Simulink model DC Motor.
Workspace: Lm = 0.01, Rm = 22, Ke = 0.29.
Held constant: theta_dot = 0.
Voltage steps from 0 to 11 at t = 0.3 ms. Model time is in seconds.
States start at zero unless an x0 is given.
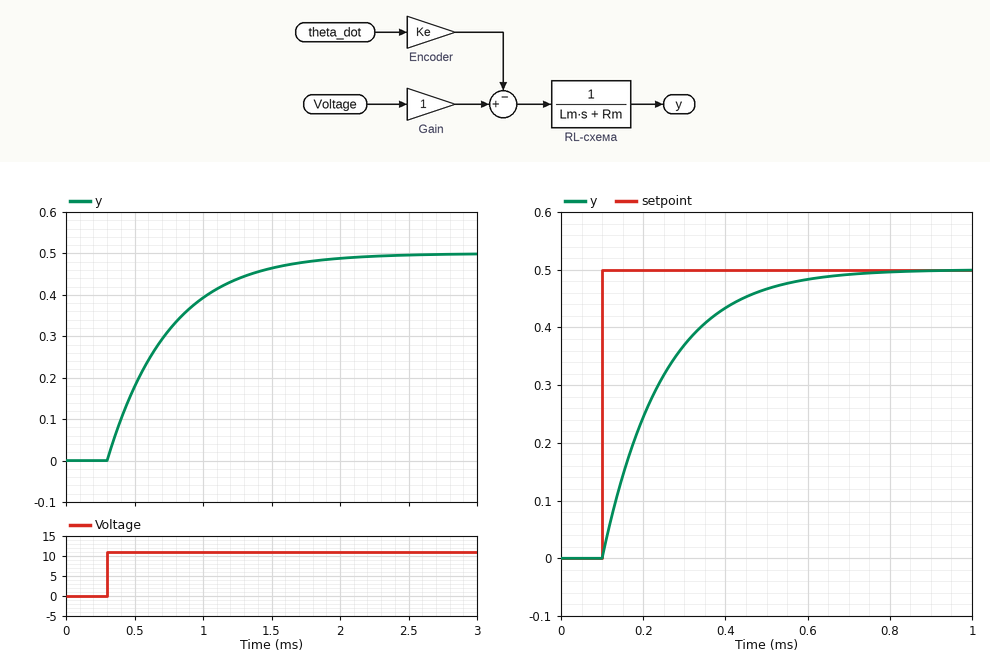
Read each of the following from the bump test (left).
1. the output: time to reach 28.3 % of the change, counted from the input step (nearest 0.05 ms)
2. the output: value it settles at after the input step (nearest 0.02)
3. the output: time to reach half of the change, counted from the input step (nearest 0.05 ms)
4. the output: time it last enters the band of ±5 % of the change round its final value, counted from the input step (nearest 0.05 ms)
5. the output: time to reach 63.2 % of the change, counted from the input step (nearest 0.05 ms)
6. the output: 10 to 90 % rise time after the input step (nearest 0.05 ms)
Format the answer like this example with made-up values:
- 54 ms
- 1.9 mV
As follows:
- 0.15 ms
- 0.50
- 0.30 ms
- 1.35 ms
- 0.45 ms
- 1.00 ms
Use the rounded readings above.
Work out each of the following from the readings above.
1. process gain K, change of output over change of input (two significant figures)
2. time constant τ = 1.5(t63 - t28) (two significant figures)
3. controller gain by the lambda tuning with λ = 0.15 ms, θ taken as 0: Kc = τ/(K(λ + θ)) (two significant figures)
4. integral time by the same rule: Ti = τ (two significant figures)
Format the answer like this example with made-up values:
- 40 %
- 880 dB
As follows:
- 0.045
- 0.45 ms
- 67
- 0.45 ms
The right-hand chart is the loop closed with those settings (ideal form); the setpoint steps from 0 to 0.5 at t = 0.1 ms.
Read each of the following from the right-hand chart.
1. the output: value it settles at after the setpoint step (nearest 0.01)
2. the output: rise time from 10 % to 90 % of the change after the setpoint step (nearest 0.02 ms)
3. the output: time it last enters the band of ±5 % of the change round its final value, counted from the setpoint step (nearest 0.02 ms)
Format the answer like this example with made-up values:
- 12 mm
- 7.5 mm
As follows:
- 0.50
- 0.32 ms
- 0.44 ms
